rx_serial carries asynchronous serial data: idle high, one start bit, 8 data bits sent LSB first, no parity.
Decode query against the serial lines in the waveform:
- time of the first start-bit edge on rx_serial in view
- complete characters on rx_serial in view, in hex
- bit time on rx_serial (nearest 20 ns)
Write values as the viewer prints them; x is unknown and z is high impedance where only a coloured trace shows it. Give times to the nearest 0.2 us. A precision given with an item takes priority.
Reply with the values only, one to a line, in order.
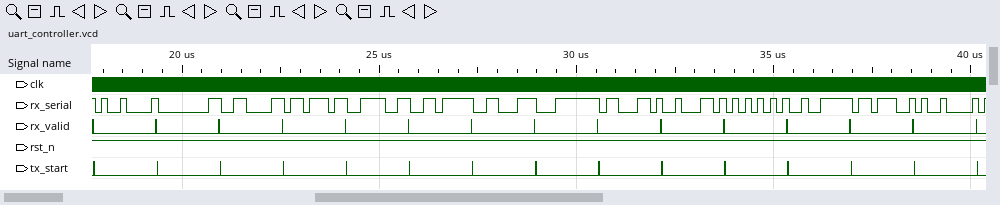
17.8 us
09, 80, 86, BB, 9E, F6, C6, FC, 63, 62, 55, F2, 3B, 09
160 ns
